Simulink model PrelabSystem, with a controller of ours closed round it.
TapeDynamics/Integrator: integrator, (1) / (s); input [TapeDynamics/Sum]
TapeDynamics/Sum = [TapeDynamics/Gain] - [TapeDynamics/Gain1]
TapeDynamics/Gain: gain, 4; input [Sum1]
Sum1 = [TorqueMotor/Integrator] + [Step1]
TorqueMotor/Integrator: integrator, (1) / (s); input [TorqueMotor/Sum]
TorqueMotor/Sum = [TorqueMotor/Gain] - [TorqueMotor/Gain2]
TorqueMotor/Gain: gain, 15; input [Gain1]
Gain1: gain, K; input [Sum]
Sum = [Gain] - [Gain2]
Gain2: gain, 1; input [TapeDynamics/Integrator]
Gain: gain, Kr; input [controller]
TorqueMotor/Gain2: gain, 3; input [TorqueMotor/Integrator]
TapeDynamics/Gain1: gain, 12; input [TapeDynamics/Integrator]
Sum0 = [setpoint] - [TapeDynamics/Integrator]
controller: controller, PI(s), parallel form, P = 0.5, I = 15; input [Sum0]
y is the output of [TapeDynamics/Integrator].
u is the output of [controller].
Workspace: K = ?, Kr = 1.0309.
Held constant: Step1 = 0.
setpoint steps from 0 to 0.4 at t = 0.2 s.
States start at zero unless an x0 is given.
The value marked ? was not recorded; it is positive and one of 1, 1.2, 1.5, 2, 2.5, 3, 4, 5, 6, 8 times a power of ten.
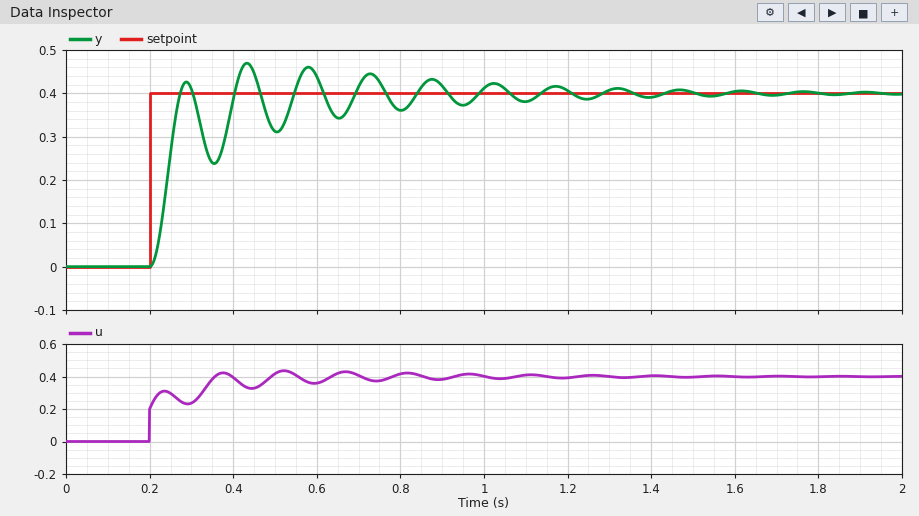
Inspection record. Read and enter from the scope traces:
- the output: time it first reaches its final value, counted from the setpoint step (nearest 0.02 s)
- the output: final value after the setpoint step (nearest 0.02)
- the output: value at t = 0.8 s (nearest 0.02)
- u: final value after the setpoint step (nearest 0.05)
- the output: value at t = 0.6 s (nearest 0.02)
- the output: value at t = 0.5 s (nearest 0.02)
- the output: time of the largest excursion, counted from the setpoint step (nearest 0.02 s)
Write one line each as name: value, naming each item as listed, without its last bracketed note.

the output: time it first reaches its final value, counted from the setpoint step: 0.08 s
the output: final value after the setpoint step: 0.40
the output: value at t = 0.8 s: 0.36
u: final value after the setpoint step: 0.40
the output: value at t = 0.6 s: 0.44
the output: value at t = 0.5 s: 0.32
the output: time of the largest excursion, counted from the setpoint step: 0.24 s
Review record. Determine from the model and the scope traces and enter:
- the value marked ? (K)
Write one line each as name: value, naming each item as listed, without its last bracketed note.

the value marked ?: 20
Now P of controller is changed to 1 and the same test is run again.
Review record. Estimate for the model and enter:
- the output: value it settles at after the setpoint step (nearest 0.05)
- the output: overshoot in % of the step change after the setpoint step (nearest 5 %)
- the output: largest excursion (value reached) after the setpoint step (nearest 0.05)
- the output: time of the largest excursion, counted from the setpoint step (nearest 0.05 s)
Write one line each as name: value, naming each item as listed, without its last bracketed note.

the output: value it settles at after the setpoint step: 0.40
the output: overshoot in % of the step change after the setpoint step: 15 %
the output: largest excursion (value reached) after the setpoint step: 0.45
the output: time of the largest excursion, counted from the setpoint step: 0.20 s
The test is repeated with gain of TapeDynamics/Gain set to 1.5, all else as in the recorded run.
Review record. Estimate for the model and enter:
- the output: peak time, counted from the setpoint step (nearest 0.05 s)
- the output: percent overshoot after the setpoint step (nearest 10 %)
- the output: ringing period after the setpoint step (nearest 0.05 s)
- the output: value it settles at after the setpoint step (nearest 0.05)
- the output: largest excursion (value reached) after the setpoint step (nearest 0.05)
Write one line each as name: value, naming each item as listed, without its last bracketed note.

the output: peak time, counted from the setpoint step: 0.15 s
the output: percent overshoot after the setpoint step: 20 %
the output: ringing period after the setpoint step: 0.25 s
the output: value it settles at after the setpoint step: 0.40
the output: largest excursion (value reached) after the setpoint step: 0.50
